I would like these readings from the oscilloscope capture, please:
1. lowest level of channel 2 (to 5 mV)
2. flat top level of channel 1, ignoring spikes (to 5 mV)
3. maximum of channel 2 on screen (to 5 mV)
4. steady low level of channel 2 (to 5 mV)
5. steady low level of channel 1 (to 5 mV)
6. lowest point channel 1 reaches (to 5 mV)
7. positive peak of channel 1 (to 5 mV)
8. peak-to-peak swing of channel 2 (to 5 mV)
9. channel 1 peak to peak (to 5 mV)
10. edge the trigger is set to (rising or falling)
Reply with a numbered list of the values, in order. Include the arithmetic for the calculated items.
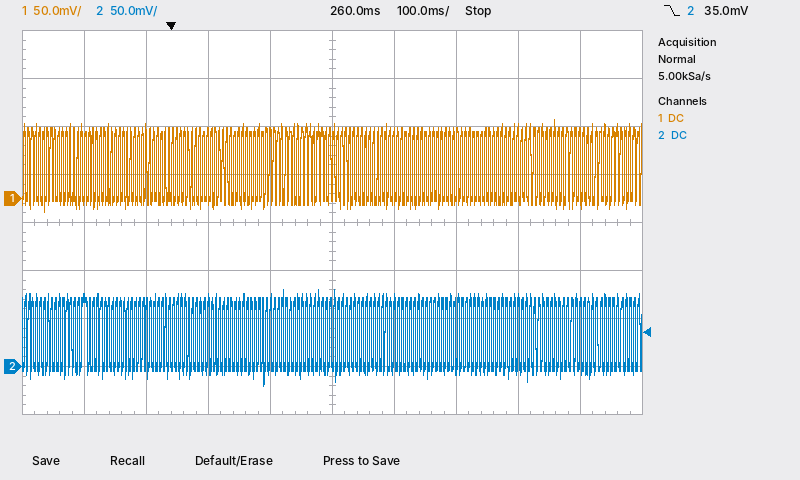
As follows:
1. -20 mV
2. 70 mV
3. 80 mV
4. 0 mV
5. 0 mV
6. -15 mV
7. 80 mV
8. 80 mV − (-20 mV) = 100 mV
9. 80 mV − (-15 mV) = 95 mV
10. falling
